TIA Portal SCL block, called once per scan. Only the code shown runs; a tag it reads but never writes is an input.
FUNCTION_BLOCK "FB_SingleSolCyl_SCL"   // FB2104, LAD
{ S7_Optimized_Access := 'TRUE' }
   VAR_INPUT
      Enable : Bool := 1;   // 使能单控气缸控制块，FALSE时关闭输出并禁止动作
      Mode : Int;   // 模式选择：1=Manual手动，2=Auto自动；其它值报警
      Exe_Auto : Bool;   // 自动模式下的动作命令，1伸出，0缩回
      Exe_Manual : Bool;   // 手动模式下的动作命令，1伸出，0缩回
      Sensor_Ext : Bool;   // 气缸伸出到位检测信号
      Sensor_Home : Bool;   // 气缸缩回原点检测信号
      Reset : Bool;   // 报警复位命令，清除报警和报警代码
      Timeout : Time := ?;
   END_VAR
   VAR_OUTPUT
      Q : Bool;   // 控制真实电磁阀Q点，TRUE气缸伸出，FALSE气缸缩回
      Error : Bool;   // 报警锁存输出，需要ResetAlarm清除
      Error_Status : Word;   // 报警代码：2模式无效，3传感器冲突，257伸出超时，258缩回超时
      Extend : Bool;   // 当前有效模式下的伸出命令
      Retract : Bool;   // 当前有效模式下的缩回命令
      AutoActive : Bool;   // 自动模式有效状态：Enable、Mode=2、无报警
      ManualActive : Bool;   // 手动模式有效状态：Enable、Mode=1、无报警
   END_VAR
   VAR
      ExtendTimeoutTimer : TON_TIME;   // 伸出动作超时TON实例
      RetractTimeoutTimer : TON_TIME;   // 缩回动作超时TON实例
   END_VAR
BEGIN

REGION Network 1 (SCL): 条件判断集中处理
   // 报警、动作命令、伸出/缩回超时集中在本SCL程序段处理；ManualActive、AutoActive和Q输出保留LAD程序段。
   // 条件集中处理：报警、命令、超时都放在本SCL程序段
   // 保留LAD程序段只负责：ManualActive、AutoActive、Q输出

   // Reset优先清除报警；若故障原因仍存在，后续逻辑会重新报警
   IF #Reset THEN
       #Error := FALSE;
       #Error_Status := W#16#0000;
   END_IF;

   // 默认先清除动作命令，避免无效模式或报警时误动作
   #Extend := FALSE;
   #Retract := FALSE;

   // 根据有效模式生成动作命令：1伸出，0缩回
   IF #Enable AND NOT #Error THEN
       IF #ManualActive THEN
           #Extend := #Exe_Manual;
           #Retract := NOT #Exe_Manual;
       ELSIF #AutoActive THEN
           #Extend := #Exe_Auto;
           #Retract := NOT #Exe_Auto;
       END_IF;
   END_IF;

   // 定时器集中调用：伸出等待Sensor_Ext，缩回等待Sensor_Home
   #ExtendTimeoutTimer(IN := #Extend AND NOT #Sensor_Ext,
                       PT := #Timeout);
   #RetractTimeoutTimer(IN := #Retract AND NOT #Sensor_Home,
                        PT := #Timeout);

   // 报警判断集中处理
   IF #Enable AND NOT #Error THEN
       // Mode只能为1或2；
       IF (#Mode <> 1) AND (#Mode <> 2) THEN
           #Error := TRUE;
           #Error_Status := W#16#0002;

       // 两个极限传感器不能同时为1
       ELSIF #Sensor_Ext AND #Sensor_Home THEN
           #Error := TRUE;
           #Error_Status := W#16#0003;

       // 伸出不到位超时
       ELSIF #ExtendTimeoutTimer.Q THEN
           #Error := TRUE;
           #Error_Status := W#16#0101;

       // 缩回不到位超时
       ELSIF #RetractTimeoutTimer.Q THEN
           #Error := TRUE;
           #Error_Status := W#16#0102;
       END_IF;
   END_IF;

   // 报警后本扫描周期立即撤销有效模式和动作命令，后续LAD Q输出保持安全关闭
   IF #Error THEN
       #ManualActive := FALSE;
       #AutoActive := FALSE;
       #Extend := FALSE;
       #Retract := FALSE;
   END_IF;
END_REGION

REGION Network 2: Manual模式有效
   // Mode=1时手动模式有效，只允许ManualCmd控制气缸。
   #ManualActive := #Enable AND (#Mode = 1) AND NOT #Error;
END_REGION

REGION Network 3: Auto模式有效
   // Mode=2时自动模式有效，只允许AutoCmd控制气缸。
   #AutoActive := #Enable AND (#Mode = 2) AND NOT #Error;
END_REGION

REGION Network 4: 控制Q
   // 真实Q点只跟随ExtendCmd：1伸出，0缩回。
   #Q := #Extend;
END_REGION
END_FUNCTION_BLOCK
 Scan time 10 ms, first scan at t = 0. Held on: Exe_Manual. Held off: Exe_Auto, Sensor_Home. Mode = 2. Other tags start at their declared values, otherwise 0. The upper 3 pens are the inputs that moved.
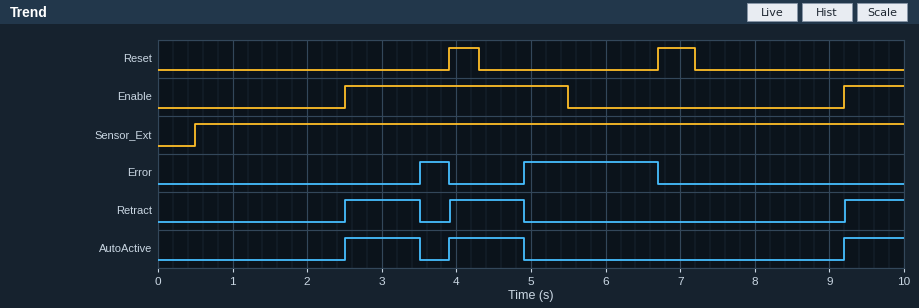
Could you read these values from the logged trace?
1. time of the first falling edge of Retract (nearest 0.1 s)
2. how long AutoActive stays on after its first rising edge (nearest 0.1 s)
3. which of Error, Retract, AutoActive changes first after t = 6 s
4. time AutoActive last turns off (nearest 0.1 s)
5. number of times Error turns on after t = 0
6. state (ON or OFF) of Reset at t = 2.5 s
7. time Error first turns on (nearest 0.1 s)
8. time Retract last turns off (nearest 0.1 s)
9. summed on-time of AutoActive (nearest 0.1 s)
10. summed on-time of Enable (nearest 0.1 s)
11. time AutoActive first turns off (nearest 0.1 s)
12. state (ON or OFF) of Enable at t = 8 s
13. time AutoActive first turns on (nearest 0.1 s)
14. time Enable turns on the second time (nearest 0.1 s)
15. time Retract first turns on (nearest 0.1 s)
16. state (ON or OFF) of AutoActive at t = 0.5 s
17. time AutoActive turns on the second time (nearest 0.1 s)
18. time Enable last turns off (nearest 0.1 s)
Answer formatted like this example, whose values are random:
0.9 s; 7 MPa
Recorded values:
3.5 s; 1.0 s; Error; 4.9 s; 2; OFF; 3.5 s; 4.9 s; 2.8 s; 3.8 s; 3.5 s; OFF; 2.5 s; 9.2 s; 2.5 s; OFF; 3.9 s; 5.5 s
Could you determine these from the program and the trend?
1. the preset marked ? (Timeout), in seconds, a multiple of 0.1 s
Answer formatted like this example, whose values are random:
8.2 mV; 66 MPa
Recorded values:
1.0 s
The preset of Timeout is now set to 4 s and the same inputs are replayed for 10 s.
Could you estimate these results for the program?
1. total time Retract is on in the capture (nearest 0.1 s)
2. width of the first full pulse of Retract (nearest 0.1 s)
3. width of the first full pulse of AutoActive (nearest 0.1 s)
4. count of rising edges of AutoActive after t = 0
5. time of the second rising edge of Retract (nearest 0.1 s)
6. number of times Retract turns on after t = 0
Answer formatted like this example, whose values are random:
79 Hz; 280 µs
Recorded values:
3.8 s; 3.0 s; 3.0 s; 2; 9.2 s; 2
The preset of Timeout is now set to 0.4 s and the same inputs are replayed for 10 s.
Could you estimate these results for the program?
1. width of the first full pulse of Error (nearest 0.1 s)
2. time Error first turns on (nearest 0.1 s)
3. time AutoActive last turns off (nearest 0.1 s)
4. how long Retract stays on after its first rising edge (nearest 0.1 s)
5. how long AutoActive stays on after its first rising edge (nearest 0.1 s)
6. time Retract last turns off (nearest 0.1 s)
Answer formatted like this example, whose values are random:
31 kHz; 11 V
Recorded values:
1.0 s; 2.9 s; 9.6 s; 0.4 s; 0.4 s; 9.6 s
